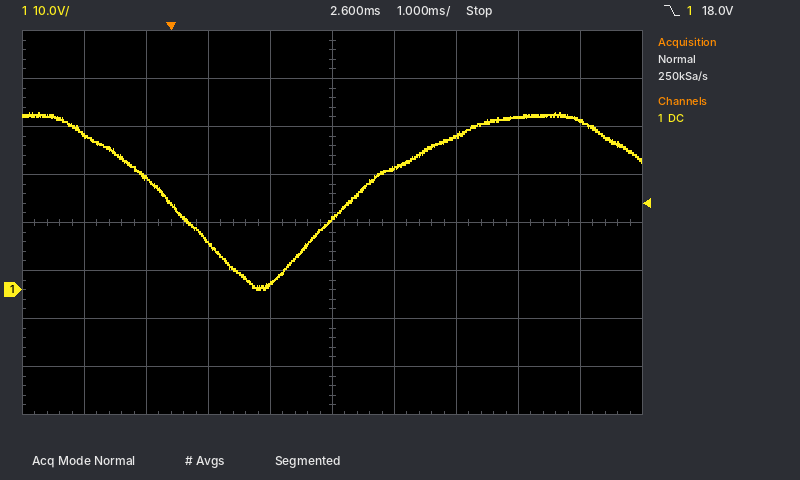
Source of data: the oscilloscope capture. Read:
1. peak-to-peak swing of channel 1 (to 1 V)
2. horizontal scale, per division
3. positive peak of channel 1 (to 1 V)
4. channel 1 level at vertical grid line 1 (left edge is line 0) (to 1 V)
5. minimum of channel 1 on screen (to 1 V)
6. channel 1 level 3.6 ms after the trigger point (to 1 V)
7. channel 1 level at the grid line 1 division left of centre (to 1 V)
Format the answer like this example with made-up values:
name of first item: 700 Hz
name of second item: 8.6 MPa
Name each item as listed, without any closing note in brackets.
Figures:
peak-to-peak swing of channel 1: 37 V
horizontal scale, per division: 1 ms
positive peak of channel 1: 37 V
channel 1 level at vertical grid line 1 (left edge is line 0): 32 V
minimum of channel 1 on screen: 0 V
channel 1 level 3.6 ms after the trigger point: 25 V
channel 1 level at the grid line 1 division left of centre: 1 V
